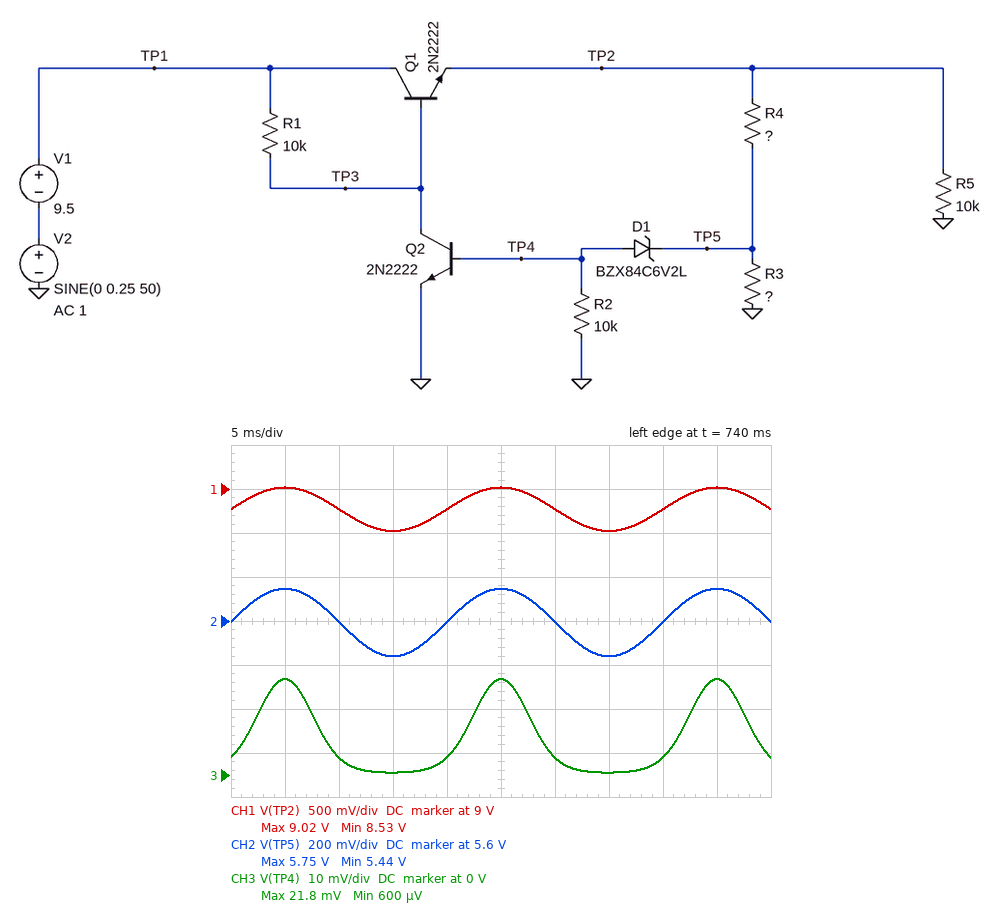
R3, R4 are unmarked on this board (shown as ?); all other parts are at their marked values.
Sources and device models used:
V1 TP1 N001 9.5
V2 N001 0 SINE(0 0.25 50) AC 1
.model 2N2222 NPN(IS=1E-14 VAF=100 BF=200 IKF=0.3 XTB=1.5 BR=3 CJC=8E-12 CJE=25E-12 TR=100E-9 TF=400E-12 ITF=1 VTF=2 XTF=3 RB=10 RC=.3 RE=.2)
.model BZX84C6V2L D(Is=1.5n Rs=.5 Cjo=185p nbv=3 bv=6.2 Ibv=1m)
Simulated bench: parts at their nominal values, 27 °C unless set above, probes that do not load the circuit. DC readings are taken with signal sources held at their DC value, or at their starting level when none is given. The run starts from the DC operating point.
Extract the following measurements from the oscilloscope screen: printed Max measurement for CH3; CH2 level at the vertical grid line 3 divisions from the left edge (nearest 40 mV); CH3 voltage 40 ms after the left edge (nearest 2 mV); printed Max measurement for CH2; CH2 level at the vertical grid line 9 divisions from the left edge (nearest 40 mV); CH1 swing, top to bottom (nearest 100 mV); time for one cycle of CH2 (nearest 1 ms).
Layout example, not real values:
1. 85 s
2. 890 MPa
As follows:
1. 21.8 mV
2. 5.44 V
3. 4 mV
4. 5.75 V
5. 5.76 V
6. 500 mV
7. 20 ms
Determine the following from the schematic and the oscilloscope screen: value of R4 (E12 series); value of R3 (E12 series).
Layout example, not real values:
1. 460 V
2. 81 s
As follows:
1. 6.8 kΩ
2. 12 kΩ
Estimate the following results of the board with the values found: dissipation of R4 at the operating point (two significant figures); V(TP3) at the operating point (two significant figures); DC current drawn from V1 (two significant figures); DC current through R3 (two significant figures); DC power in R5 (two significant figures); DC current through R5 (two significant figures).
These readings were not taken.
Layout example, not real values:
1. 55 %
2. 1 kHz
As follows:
1. 1.5 mW
2. 9.4 V
3. 1.3 mA
4. 470 µA
5. 7.7 mW
6. 880 µA
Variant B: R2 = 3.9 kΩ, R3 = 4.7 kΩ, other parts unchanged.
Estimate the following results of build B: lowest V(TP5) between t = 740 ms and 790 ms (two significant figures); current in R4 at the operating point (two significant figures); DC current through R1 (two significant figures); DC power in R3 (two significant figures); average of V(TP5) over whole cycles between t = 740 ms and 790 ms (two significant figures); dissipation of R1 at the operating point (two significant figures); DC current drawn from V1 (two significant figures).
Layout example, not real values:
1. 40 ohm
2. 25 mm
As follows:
1. 3.5 V
2. 760 µA
3. 8.2 µA
4. 2.7 mW
5. 3.6 V
6. 670 nW
7. 1.6 mA
